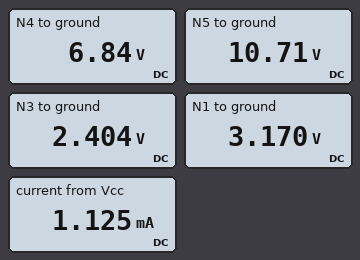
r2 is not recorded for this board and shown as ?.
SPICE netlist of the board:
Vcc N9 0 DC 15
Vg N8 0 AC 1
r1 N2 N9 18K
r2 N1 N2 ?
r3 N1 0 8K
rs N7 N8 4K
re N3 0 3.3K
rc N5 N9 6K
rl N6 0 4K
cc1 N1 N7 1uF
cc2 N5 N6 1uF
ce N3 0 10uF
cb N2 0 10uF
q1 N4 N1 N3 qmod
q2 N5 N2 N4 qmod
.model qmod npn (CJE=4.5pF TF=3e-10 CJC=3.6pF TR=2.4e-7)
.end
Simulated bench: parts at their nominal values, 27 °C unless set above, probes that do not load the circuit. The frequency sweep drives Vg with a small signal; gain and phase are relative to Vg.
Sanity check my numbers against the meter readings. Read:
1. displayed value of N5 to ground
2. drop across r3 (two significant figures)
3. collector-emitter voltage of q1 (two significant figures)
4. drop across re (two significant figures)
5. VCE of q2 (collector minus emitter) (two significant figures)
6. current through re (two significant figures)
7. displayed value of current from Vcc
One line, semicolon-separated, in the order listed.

10.71 V; 3.2 V; 4.4 V; 2.4 V; 3.9 V; 730 µA; 1.125 mA
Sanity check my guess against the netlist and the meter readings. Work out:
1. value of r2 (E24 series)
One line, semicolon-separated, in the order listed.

11 kΩ
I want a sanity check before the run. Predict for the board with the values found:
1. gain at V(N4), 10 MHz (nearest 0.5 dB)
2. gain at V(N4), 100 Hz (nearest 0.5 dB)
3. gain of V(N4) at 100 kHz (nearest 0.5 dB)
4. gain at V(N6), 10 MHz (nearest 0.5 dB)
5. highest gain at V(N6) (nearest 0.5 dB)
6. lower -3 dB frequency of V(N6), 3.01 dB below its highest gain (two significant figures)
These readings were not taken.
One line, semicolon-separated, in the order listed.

-15.5 dB; -19.0 dB; -9.5 dB; 20.5 dB; 27.0 dB; 300 Hz
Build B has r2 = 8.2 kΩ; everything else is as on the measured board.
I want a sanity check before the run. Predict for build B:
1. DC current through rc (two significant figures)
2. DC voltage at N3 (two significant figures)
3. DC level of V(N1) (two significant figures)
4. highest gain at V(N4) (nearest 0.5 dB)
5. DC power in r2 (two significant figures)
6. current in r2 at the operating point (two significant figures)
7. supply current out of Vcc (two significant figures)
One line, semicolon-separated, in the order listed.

790 µA; 2.7 V; 3.4 V; -10.0 dB; 1.6 mW; 440 µA; 1.2 mA
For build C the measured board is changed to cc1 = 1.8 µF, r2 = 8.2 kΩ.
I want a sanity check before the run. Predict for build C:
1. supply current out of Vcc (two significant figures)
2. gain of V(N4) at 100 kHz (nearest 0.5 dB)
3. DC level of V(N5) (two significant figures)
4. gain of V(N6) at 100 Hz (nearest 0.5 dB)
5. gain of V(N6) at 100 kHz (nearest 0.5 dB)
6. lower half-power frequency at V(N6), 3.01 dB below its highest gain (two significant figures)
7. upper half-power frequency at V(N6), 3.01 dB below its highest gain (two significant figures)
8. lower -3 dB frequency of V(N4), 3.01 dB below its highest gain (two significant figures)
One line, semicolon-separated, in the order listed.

1.2 mA; -10.0 dB; 10 V; 16.5 dB; 27.0 dB; 320 Hz; 5.8 MHz; 310 Hz
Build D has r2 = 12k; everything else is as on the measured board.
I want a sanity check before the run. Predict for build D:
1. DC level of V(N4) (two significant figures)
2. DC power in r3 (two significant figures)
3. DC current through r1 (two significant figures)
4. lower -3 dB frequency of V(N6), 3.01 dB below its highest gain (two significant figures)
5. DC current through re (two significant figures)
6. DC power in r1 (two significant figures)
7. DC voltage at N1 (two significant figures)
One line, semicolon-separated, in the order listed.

7.0 V; 1.2 mW; 400 µA; 290 Hz; 700 µA; 2.9 mW; 3.1 V
